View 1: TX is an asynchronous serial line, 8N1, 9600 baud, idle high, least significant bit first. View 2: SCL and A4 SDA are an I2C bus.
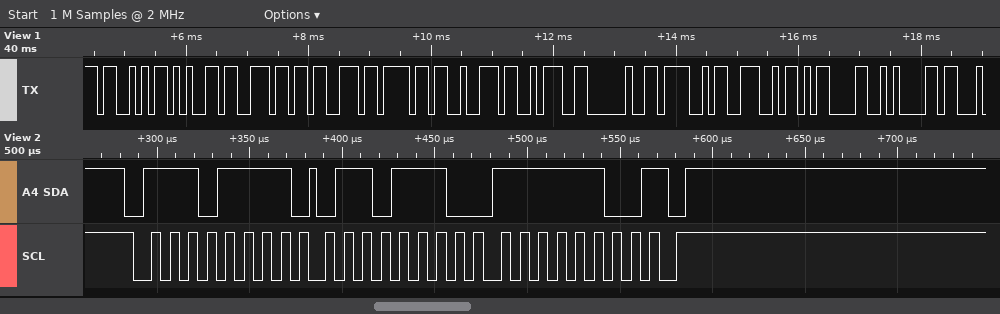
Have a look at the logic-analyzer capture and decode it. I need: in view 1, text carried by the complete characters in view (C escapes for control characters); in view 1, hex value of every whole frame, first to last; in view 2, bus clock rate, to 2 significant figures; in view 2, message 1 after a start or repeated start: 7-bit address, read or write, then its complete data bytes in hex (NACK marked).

"Sensor: ON\r\n"
0x53 0x65 0x6E 0x73 0x6F 0x72 0x3A 0x20 0x4F 0x4E 0x0D 0x0A
100 kHz
0x77 read: 6E FC NACK
